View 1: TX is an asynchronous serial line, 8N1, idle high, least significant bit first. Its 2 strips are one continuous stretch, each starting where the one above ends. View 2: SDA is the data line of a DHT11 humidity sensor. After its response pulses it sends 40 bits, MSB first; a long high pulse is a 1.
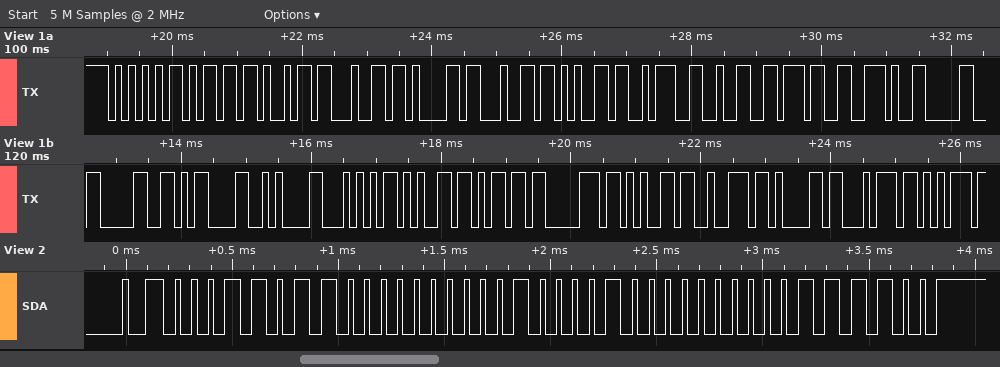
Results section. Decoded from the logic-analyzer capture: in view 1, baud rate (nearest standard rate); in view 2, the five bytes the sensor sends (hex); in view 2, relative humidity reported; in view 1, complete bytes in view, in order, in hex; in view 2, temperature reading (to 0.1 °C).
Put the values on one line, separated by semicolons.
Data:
9600 baud; 1B 00 21 00 3C; 27 %; 55 6D 69 64 61 64 65 3A 32 37 2E 30 30 0D 0A 54 65 6D 70 65 72 61 74 75; 33.0 °C
